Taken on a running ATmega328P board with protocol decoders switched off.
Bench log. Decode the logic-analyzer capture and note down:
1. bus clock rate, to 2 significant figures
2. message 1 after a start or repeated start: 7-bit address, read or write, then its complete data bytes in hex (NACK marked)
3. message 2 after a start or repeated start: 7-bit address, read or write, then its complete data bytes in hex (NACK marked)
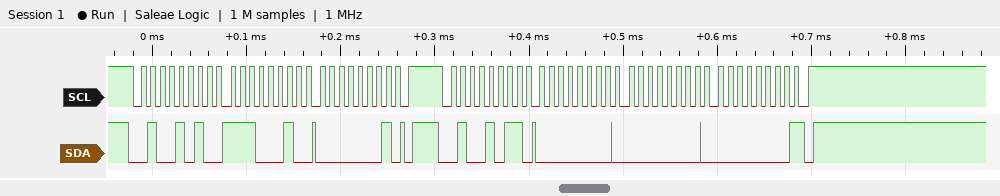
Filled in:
100 kHz
0x25 write: E2 01
0x25 read: 00 00 00 NACK
